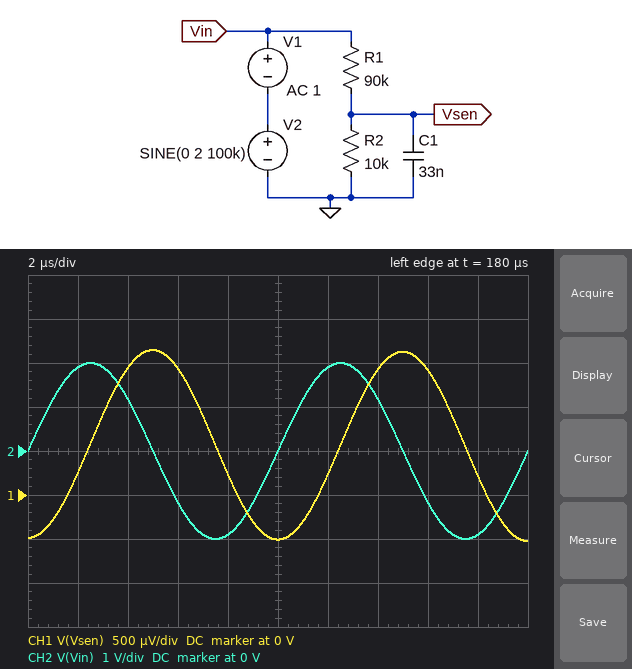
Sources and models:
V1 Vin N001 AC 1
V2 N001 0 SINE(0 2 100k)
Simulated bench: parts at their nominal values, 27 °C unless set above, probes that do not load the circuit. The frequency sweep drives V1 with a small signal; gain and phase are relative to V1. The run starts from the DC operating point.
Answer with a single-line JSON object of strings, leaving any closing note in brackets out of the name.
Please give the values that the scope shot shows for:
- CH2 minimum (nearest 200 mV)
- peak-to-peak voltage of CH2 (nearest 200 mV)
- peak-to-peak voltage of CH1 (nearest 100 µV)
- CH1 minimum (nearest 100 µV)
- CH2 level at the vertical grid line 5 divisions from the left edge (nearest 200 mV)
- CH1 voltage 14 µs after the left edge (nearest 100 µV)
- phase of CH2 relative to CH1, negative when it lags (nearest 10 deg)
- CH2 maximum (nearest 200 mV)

{"CH2 minimum": "-2.0 V", "peak-to-peak voltage of CH2": "4.0 V", "peak-to-peak voltage of CH1": "2.2 mV", "CH1 minimum": "-500 µV", "CH2 level at the vertical grid line 5 divisions from the left edge": "0 V", "CH1 voltage 14 µs after the left edge": "1.4 mV", "phase of CH2 relative to CH1, negative when it lags": "90 deg", "CH2 maximum": "2.0 V"}
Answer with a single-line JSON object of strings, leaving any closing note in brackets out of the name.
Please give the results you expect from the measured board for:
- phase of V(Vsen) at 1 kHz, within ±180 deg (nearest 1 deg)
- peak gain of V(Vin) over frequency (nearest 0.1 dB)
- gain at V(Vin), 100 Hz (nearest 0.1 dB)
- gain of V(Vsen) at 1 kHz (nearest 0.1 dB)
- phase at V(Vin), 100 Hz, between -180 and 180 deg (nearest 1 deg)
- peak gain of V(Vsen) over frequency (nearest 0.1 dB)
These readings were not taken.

{"phase of V(Vsen) at 1 kHz, within ±180 deg": "-62 deg", "peak gain of V(Vin) over frequency": "0 dB", "gain at V(Vin), 100 Hz": "0 dB", "gain of V(Vsen) at 1 kHz": "-26.5 dB", "phase at V(Vin), 100 Hz, between -180 and 180 deg": "0 deg", "peak gain of V(Vsen) over frequency": "-20.0 dB"}
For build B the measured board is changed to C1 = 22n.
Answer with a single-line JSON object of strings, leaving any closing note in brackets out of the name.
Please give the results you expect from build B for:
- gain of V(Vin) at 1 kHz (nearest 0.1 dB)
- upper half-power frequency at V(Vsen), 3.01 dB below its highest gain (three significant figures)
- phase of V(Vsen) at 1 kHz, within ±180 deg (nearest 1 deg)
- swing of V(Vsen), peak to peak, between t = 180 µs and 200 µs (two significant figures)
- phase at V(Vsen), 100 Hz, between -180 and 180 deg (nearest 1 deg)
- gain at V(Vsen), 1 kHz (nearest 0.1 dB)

{"gain of V(Vin) at 1 kHz": "0 dB", "upper half-power frequency at V(Vsen), 3.01 dB below its highest gain": "804 Hz", "phase of V(Vsen) at 1 kHz, within ±180 deg": "-51 deg", "swing of V(Vsen), peak to peak, between t = 180 µs and 200 µs": "3.3 mV", "phase at V(Vsen), 100 Hz, between -180 and 180 deg": "-7 deg", "gain at V(Vsen), 1 kHz": "-24.1 dB"}
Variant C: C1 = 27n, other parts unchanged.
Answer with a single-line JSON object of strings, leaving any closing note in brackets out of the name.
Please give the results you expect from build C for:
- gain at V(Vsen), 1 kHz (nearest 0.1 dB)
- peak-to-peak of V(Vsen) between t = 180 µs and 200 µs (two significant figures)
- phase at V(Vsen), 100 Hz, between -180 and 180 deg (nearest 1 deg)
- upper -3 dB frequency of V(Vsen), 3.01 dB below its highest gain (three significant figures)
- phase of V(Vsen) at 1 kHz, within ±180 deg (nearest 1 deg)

{"gain at V(Vsen), 1 kHz": "-25.2 dB", "peak-to-peak of V(Vsen) between t = 180 µs and 200 µs": "2.7 mV", "phase at V(Vsen), 100 Hz, between -180 and 180 deg": "-9 deg", "upper -3 dB frequency of V(Vsen), 3.01 dB below its highest gain": "655 Hz", "phase of V(Vsen) at 1 kHz, within ±180 deg": "-57 deg"}
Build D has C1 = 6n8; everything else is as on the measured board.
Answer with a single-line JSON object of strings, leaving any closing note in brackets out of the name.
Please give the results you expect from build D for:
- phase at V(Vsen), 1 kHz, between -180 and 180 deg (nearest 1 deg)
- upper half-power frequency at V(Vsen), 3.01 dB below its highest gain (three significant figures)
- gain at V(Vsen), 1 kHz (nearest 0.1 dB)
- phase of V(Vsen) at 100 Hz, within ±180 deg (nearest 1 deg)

{"phase at V(Vsen), 1 kHz, between -180 and 180 deg": "-21 deg", "upper half-power frequency at V(Vsen), 3.01 dB below its highest gain": "2.60 kHz", "gain at V(Vsen), 1 kHz": "-20.6 dB", "phase of V(Vsen) at 100 Hz, within ±180 deg": "-2 deg"}
